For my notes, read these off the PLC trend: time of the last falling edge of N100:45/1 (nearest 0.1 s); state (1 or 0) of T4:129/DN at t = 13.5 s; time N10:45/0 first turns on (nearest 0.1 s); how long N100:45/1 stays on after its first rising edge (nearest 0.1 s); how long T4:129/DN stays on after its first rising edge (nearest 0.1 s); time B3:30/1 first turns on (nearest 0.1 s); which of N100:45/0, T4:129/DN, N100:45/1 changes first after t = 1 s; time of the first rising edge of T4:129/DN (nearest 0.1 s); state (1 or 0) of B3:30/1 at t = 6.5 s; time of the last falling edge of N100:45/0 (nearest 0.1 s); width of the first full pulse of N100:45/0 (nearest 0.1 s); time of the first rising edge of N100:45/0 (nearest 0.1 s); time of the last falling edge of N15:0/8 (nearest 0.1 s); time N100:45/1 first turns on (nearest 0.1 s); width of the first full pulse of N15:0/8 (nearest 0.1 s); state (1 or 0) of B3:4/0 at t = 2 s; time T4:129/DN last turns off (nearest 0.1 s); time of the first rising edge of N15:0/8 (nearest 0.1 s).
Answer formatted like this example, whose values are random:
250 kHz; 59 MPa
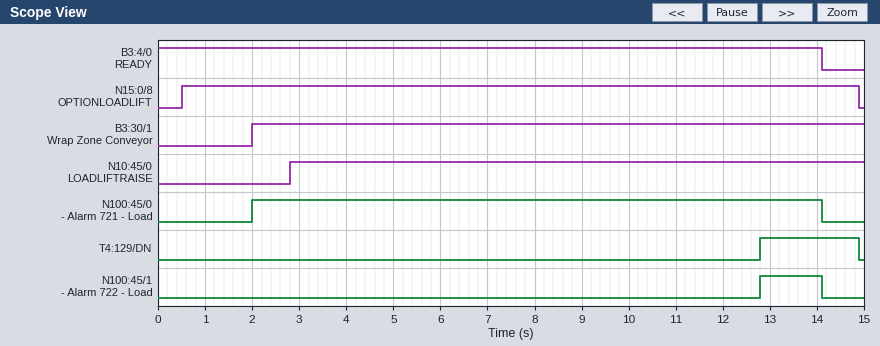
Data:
14.1 s; 1; 2.8 s; 1.3 s; 2.1 s; 2.0 s; N100:45/0; 12.8 s; 1; 14.1 s; 12.1 s; 2.0 s; 14.9 s; 12.8 s; 14.4 s; 1; 14.9 s; 0.5 s
